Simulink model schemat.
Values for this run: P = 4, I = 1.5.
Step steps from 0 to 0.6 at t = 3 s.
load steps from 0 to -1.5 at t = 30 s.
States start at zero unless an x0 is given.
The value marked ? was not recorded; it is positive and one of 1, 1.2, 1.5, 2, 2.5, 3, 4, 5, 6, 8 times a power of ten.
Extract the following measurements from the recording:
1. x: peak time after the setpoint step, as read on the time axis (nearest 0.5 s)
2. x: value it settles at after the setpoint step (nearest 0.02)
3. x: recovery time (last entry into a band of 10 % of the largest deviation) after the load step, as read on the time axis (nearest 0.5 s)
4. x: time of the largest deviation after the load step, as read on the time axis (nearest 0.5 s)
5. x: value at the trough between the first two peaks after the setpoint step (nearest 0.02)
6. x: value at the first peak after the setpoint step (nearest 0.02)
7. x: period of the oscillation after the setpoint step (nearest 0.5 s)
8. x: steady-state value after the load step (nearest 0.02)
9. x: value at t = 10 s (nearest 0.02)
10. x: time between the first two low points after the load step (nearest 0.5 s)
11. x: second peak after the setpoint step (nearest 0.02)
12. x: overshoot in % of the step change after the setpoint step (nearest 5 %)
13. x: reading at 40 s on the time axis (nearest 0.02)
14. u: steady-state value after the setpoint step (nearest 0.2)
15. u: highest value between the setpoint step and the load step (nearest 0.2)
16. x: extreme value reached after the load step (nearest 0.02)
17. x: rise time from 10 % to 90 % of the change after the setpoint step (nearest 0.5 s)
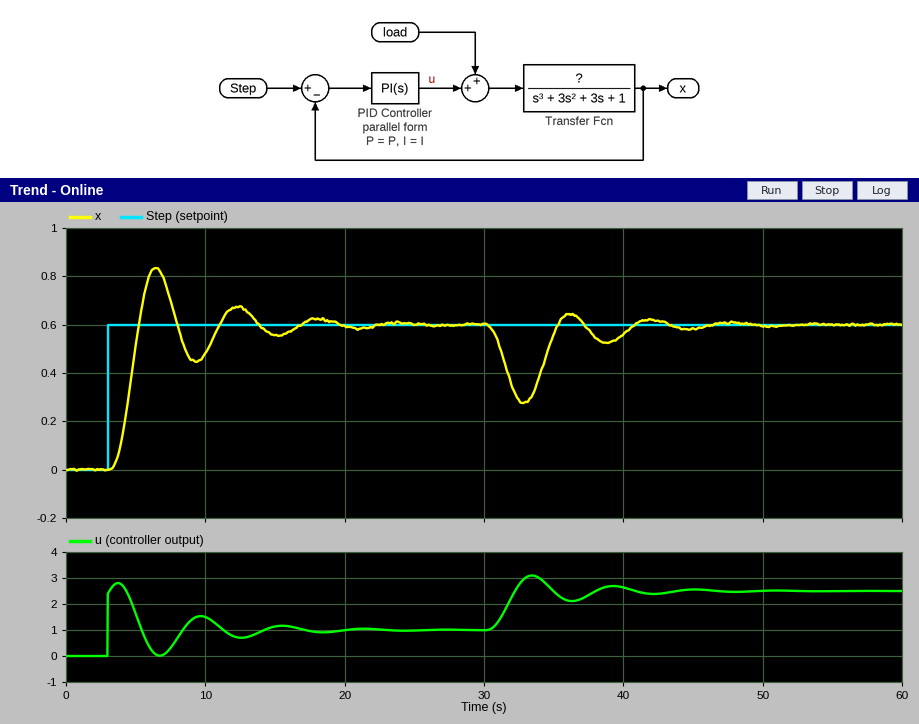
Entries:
6.5 s
0.60
40.0 s
33.0 s
0.44
0.84
6.0 s
0.60
0.48
6.0 s
0.68
40 %
0.56
1.0
2.8
0.28
1.5 s
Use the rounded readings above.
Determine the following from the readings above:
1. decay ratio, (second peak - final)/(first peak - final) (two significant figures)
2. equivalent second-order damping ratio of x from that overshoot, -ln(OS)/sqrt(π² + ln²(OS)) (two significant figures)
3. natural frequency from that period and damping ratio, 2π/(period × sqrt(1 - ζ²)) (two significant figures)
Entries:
0.33
0.28
1.1 rad/s
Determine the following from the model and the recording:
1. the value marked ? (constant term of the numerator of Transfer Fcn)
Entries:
0.6
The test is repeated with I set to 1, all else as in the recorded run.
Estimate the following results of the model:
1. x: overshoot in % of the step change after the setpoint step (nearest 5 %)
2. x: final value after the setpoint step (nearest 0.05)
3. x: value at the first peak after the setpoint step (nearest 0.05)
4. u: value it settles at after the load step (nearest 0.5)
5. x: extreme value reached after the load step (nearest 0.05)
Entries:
25 %
0.60
0.75
2.5
0.25
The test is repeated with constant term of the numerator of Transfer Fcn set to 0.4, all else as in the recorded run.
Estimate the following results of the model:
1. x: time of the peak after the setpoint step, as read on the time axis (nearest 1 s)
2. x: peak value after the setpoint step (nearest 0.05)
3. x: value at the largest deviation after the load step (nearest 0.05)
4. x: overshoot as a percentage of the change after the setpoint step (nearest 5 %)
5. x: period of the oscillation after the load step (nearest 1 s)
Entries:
7 s
0.70
0.35
20 %
7 s
